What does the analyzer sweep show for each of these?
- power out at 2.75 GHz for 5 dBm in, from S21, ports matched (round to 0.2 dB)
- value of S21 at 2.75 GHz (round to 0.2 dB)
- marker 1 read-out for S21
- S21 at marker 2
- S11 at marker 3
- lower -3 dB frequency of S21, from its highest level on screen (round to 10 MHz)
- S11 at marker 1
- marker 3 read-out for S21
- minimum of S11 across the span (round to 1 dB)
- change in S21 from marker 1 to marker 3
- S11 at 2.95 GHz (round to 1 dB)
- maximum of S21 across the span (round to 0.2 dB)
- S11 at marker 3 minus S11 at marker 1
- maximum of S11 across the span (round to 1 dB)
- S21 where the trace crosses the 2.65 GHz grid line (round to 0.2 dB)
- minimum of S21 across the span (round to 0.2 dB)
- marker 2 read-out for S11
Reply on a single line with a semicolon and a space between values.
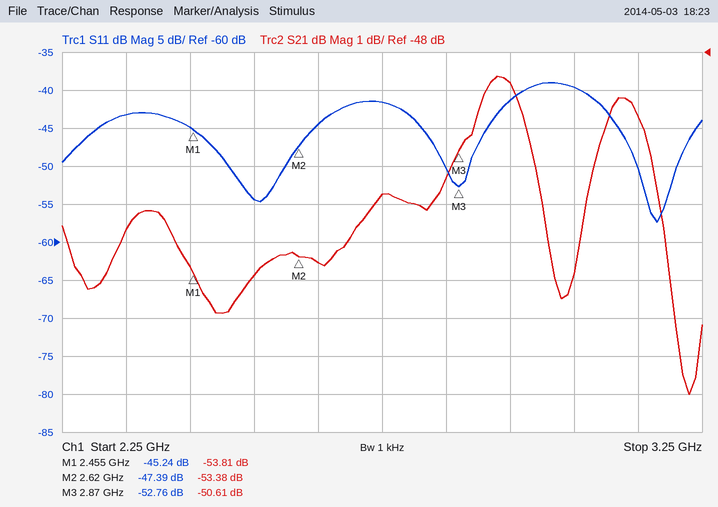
-46.8 dBm; -51.8 dB; -53.81 dB; -53.38 dB; -52.76 dB; 2.84 GHz; -45.24 dB; -50.61 dB; -57 dB; 3.20 dB; -41 dB; -48.6 dB; -7.52 dB; -39 dB; -53.6 dB; -57.0 dB; -47.39 dB
